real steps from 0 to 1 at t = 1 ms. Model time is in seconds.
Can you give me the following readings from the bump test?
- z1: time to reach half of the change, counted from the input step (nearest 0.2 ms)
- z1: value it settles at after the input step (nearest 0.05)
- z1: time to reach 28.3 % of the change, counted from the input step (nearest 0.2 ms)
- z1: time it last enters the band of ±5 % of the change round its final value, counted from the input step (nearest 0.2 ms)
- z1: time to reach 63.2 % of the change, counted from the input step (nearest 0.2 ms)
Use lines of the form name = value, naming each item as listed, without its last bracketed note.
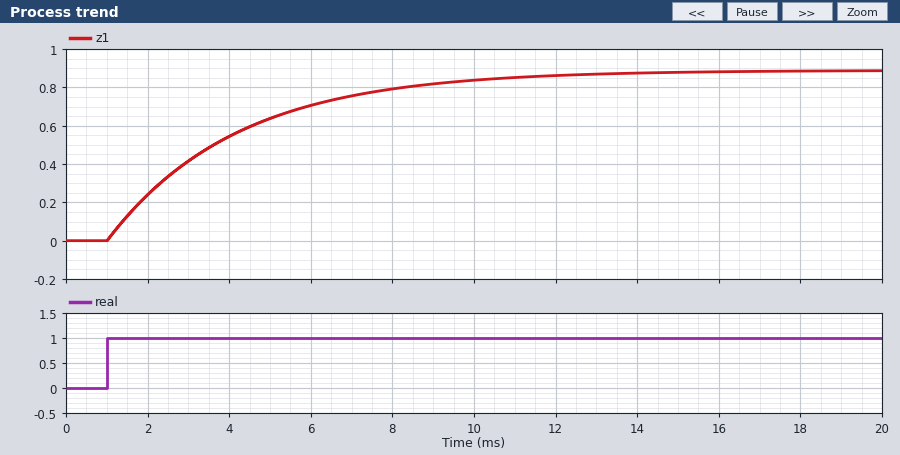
z1: time to reach half of the change, counted from the input step = 2.2 ms
z1: value it settles at after the input step = 0.90
z1: time to reach 28.3 % of the change, counted from the input step = 1.0 ms
z1: time it last enters the band of ±5 % of the change round its final value, counted from the input step = 9.4 ms
z1: time to reach 63.2 % of the change, counted from the input step = 3.2 ms
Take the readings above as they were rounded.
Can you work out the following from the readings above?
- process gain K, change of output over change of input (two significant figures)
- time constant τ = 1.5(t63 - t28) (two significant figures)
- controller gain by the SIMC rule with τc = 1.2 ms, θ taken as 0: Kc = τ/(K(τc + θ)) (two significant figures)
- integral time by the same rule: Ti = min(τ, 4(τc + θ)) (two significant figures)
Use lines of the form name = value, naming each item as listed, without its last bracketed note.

process gain K, change of output over change of input = 0.90
time constant τ = 1.5(t63 - t28) = 3.3 ms
controller gain by the SIMC rule with τc = 1.2 ms, θ taken as 0: Kc = τ/(K(τc + θ)) = 3.1
integral time by the same rule: Ti = min(τ, 4(τc + θ)) = 3.3 ms
